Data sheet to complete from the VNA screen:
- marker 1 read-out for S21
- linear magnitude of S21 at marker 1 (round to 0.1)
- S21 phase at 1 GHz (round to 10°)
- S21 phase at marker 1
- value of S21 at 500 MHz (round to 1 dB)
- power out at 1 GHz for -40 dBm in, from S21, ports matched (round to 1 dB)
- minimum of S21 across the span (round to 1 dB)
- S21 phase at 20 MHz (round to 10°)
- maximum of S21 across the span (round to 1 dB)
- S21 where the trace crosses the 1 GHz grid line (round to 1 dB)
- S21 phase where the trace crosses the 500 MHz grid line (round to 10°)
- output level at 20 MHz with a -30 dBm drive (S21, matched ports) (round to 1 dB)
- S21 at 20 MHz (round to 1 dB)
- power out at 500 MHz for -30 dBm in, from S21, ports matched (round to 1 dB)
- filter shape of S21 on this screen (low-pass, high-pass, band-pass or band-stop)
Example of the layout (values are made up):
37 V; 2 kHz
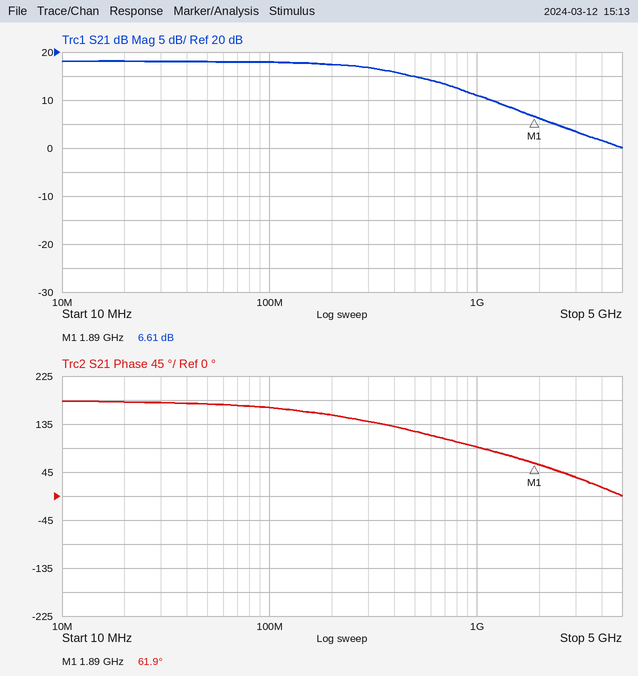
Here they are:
6.61 dB; 2.1; 90°; 61.9°; 15 dB; -29 dBm; 0 dB; 180°; 18 dB; 11 dB; 120°; -12 dBm; 18 dB; -15 dBm; low-pass
